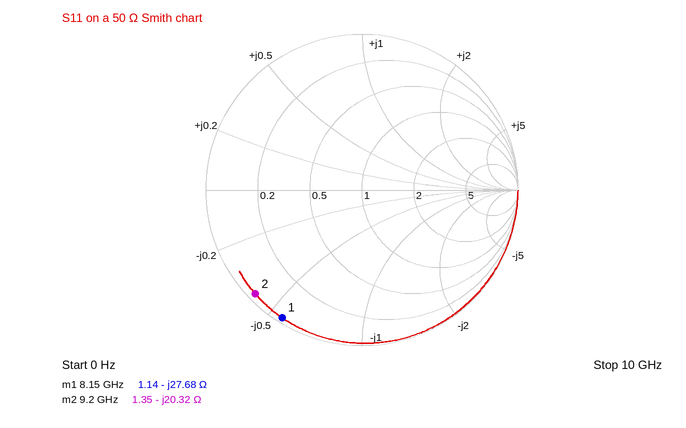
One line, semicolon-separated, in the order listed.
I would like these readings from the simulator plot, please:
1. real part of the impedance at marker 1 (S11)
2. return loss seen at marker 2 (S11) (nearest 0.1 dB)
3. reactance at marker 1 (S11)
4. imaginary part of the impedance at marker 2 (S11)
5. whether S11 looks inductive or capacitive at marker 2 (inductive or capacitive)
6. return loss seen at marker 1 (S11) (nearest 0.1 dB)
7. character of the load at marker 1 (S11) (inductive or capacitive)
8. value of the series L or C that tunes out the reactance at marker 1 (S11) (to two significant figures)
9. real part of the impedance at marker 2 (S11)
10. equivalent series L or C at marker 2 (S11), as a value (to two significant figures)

1.14 Ω; 0.4 dB; -27.68 Ω; -20.32 Ω; capacitive; 0.3 dB; capacitive; 540 pH; 1.35 Ω; 850 fF
